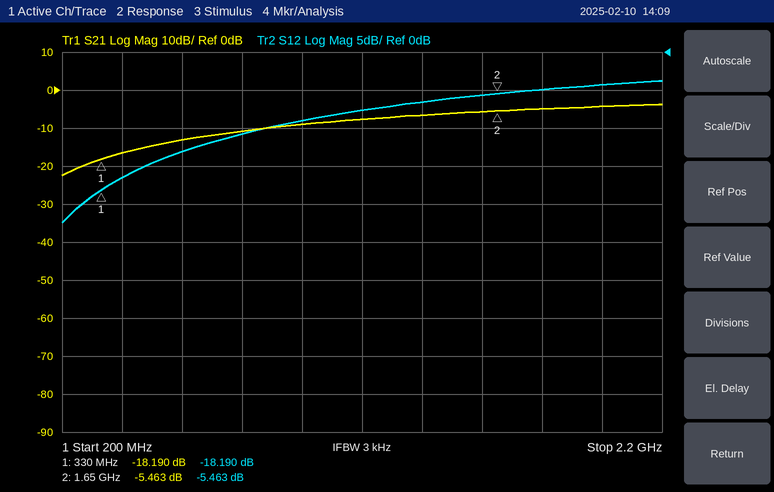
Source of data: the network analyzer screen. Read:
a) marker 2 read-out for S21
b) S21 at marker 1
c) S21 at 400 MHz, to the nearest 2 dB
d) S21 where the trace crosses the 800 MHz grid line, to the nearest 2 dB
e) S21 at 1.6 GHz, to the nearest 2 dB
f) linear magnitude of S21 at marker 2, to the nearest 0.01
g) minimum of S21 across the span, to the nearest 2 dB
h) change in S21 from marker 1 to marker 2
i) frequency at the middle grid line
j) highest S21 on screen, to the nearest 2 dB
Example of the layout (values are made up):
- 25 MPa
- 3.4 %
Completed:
- -5.463 dB
- -18.190 dB
- -16 dB
- -10 dB
- -6 dB
- 0.53
- -22 dB
- 12.727 dB
- 1.2 GHz
- -4 dB
